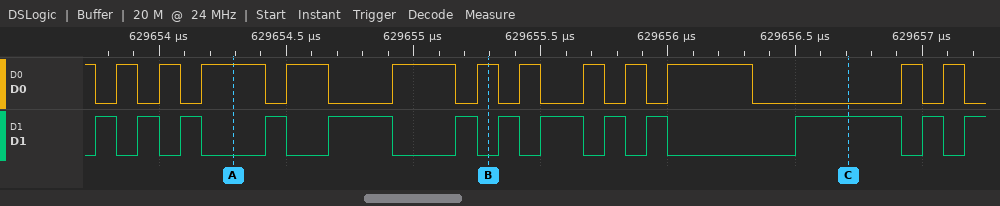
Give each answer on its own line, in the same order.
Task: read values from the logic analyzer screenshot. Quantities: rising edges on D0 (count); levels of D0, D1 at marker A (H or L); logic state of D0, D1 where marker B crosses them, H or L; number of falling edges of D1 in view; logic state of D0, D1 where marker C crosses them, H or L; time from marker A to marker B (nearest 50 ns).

12
D0=H, D1=L
D0=H, D1=L
12
D0=L, D1=H
1000 ns
